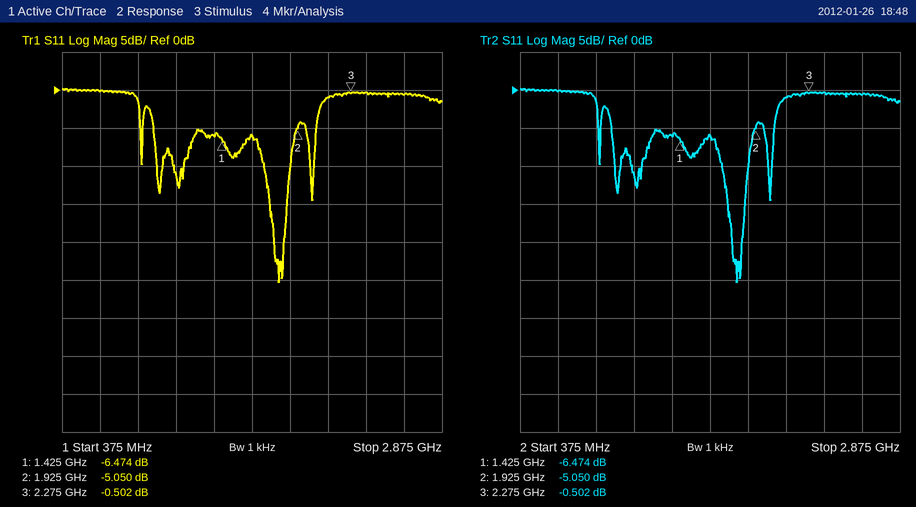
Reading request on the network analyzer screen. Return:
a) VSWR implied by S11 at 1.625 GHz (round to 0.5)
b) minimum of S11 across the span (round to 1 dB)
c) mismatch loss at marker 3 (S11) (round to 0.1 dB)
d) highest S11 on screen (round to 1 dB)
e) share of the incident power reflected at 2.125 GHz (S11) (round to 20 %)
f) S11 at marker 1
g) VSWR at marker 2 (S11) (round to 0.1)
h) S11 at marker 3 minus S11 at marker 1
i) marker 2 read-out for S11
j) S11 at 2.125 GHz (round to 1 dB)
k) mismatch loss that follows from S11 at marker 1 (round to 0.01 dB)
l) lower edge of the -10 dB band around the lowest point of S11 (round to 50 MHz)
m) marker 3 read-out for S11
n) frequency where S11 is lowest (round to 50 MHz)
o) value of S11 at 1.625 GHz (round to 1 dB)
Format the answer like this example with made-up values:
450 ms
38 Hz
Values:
3.0
-25 dB
9.6 dB
0 dB
80 %
-6.474 dB
3.5
5.972 dB
-5.050 dB
-1 dB
1.11 dB
1.70 GHz
-0.502 dB
1.80 GHz
-6 dB
